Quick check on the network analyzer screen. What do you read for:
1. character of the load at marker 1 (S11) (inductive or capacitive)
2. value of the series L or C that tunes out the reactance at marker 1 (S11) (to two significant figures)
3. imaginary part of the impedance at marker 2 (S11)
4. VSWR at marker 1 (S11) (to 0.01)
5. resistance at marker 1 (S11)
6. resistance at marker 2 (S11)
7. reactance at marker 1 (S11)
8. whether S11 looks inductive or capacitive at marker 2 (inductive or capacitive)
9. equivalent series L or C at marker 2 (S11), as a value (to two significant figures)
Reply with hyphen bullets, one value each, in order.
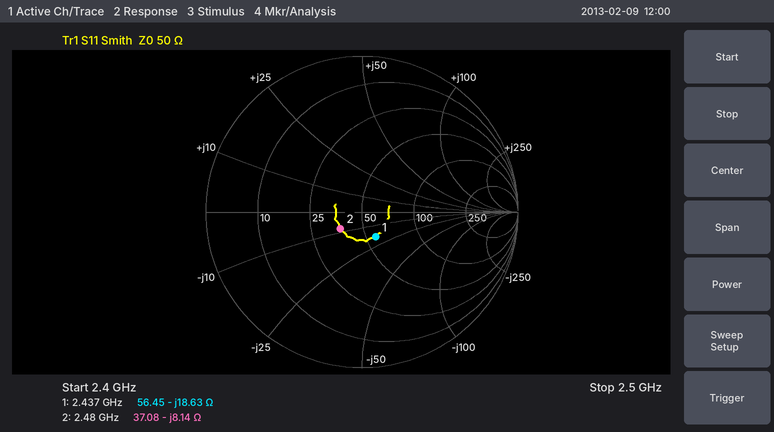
- capacitive
- 1.2 nH
- -8.14 Ω
- 1.45
- 56.45 Ω
- 37.08 Ω
- -18.63 Ω
- capacitive
- 7.9 pF
